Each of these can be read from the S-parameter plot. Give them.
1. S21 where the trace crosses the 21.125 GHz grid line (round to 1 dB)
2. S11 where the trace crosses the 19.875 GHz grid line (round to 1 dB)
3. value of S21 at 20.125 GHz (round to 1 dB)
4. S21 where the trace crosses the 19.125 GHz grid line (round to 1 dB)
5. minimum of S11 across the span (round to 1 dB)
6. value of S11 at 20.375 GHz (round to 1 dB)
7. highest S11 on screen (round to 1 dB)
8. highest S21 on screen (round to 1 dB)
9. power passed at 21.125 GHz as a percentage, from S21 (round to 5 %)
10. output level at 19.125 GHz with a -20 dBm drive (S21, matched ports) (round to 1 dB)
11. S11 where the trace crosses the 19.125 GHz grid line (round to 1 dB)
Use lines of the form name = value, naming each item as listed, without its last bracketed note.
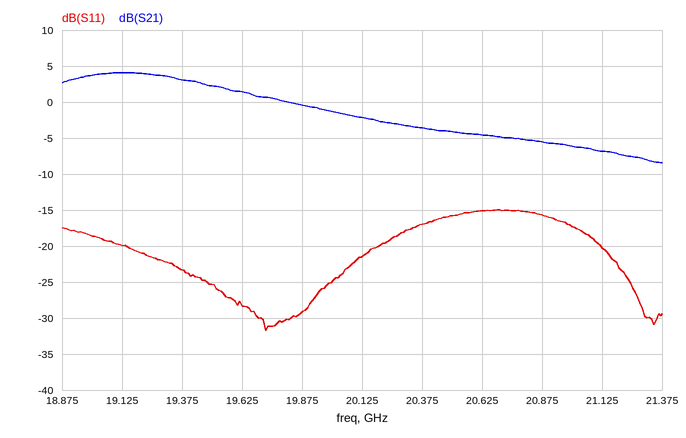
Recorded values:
S21 where the trace crosses the 21.125 GHz grid line = -7 dB
S11 where the trace crosses the 19.875 GHz grid line = -29 dB
value of S21 at 20.125 GHz = -2 dB
S21 where the trace crosses the 19.125 GHz grid line = 4 dB
minimum of S11 across the span = -32 dB
value of S11 at 20.375 GHz = -17 dB
highest S11 on screen = -15 dB
highest S21 on screen = 4 dB
power passed at 21.125 GHz as a percentage, from S21 = 20 %
output level at 19.125 GHz with a -20 dBm drive (S21, matched ports) = -16 dBm
S11 where the trace crosses the 19.125 GHz grid line = -20 dB
